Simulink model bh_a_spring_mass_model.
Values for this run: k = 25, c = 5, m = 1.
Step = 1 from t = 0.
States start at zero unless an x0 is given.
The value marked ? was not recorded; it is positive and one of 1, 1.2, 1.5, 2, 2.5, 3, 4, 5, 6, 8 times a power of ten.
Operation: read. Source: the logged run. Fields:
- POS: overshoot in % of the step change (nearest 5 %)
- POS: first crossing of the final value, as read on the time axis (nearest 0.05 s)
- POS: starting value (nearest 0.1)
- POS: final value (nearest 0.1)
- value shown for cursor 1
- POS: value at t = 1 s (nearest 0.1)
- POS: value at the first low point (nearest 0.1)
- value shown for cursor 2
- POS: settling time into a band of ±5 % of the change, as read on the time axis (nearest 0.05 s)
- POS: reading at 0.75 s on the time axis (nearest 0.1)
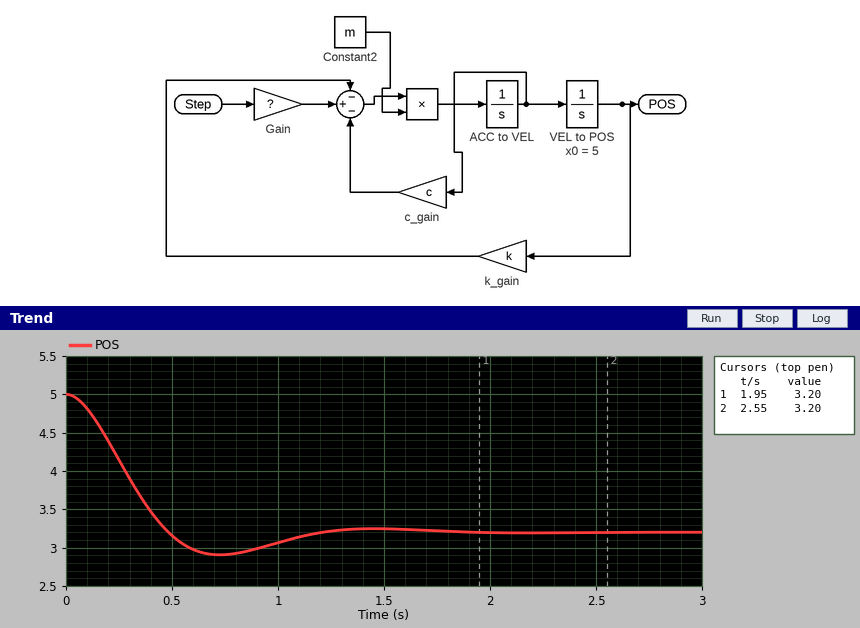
15 %
0.50 s
5.0
3.2
3.20
3.1
2.9
3.20
1.05 s
2.9
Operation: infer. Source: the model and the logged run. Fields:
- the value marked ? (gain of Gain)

80
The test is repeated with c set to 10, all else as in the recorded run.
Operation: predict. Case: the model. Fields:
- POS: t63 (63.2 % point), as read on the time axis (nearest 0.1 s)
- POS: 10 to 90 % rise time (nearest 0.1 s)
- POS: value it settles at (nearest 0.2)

0.4 s
0.7 s
3.2
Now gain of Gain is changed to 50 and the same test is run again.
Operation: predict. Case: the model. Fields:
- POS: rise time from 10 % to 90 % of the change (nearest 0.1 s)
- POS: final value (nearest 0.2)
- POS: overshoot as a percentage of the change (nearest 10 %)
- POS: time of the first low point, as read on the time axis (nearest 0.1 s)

0.3 s
2.0
20 %
0.7 s
